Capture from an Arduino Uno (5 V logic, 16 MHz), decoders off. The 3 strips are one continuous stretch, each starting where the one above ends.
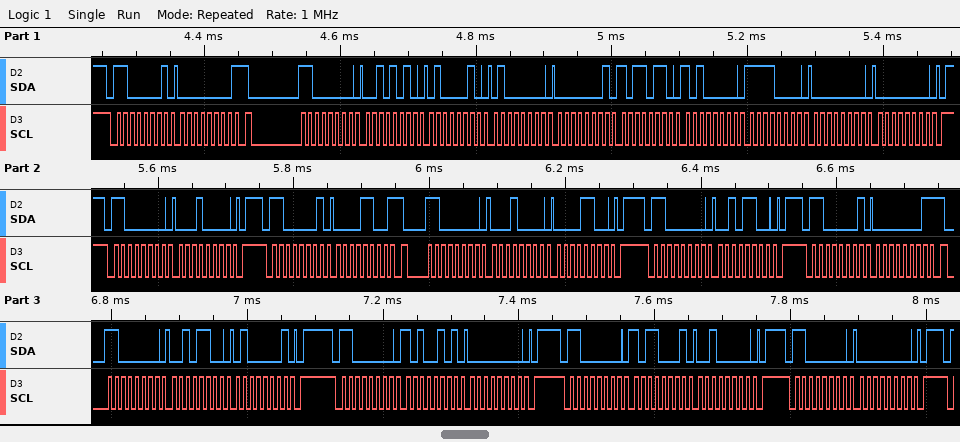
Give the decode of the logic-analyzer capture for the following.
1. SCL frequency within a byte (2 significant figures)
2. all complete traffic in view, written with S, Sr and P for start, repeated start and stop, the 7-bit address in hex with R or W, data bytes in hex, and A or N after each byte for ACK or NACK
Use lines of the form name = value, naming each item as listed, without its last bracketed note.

SCL frequency within a byte = 100 kHz
all complete traffic in view, written with S, Sr and P for start, repeated start and stop, the 7-bit address in hex with R or W, data bytes in hex, and A or N after each byte for ACK or NACK = S 60R A 00 N Sr 60W A 2A A 42 A 40 A 01 A B6 A A0 A F0 A 00 A 00 A P S 60W A 10 A P S 60R A 0C N Sr 60W A 10 A 0C A P S 60W A 2C A P S 60R A 01 N Sr 60W A 2C A 41 A P S 60W A A5 A 00 A P S 60W A B1 A 20 A P S 60W A 00 A P
